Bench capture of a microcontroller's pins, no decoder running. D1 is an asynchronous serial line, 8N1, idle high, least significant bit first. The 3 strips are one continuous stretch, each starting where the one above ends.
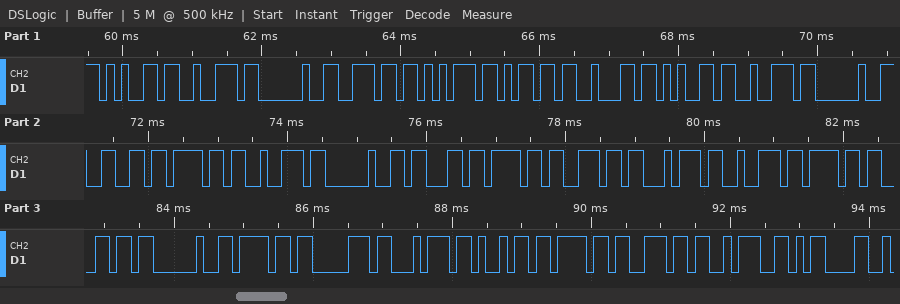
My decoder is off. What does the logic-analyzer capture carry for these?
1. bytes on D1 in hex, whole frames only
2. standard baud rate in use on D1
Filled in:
65 72 20 6E 75 6D 62 65 72 20 66 6F 72 20 63 6F 6E 74 72 6F 6C 20 6F 70 74 69 6F 6E 3A 0D
9600 baud
